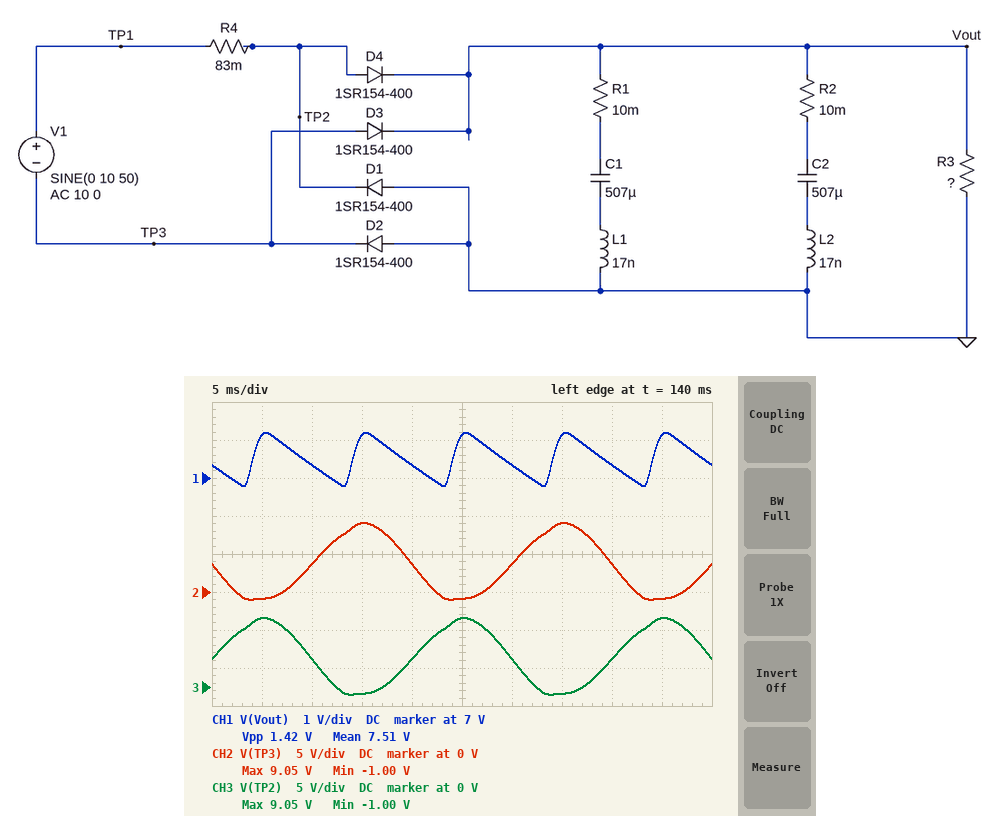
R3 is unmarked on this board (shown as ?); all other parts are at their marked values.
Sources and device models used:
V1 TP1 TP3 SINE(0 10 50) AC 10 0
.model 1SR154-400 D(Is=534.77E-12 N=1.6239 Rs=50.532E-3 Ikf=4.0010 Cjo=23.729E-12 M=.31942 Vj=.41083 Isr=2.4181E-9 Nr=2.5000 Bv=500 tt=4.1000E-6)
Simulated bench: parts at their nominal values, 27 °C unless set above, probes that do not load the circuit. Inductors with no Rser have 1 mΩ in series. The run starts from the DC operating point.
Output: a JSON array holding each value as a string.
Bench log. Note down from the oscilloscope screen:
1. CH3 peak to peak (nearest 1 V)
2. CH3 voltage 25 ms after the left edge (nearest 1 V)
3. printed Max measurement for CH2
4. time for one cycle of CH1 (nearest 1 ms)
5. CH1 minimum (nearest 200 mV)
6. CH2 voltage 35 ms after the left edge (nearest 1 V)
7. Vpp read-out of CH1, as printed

["10 V", "9 V", "9.05 V", "10 ms", "6.8 V", "9 V", "1.42 V"]
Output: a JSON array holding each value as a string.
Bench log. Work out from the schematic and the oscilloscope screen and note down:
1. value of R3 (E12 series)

["39 Ω"]
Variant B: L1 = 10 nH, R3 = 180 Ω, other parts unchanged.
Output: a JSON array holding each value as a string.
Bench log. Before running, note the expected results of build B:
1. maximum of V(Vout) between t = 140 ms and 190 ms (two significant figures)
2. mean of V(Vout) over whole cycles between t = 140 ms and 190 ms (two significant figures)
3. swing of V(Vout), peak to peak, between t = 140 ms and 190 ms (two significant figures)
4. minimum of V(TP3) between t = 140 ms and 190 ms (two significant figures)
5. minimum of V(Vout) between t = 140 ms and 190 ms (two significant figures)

["8.3 V", "8.1 V", "360 mV", "-900 mV", "7.9 V"]
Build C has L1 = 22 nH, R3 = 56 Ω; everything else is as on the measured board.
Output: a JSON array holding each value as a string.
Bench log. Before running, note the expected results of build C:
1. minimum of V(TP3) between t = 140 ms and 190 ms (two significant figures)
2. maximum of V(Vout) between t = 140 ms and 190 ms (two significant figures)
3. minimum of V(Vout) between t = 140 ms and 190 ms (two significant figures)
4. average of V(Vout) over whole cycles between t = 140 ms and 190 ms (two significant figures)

["-970 mV", "8.2 V", "7.2 V", "7.7 V"]
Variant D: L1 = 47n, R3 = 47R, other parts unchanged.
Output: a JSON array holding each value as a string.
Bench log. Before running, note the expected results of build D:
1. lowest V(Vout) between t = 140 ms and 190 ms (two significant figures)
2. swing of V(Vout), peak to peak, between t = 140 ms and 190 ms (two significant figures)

["7.0 V", "1.2 V"]
